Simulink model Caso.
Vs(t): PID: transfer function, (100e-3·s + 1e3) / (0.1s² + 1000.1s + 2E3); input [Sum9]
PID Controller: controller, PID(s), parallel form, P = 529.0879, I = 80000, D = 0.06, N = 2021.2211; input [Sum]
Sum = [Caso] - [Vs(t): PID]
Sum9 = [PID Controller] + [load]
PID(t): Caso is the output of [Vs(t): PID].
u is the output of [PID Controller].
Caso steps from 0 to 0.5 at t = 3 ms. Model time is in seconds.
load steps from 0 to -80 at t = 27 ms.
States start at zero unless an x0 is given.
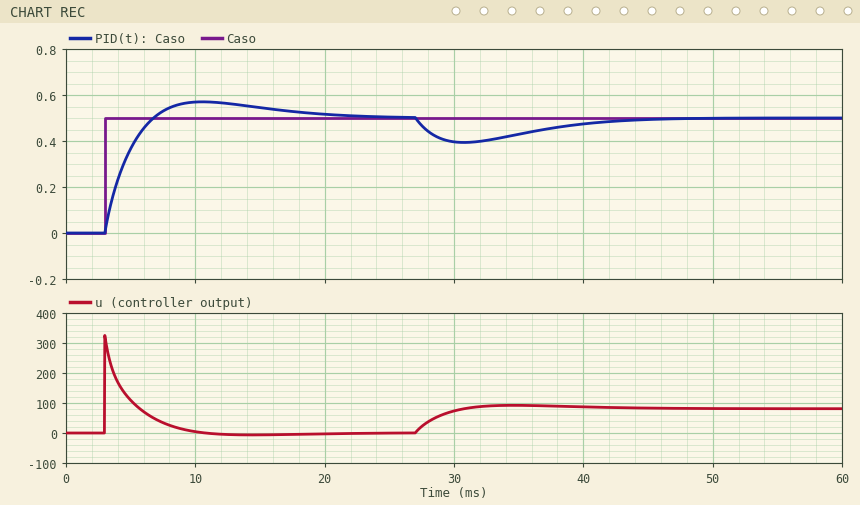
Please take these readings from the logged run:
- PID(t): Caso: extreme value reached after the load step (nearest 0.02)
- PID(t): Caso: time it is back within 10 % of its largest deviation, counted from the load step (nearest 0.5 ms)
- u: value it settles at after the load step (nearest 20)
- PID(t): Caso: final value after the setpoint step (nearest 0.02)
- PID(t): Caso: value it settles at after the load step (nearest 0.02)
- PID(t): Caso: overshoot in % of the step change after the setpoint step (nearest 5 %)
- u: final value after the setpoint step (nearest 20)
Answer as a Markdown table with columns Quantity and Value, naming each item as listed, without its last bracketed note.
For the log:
| Quantity | Value |
|---|---|
| PID(t): Caso: extreme value reached after the load step | 0.40 |
| PID(t): Caso: time it is back within 10 % of its largest deviation, counted from the load step | 16.5 ms |
| u: value it settles at after the load step | 80 |
| PID(t): Caso: final value after the setpoint step | 0.50 |
| PID(t): Caso: value it settles at after the load step | 0.50 |
| PID(t): Caso: overshoot in % of the step change after the setpoint step | 15 % |
| u: final value after the setpoint step | 0 |
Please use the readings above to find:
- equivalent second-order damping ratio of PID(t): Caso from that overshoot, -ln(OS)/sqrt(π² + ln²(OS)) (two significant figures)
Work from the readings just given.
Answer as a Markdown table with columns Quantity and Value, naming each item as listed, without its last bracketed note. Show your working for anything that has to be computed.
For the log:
| Quantity | Value |
|---|---|
| equivalent second-order damping ratio of PID(t): Caso from that overshoot, -ln(OS)/sqrt(π² + ln²(OS)) | ln(0.15) = -1.897; 1.897 / sqrt(9.870 + 3.599) = 0.52 |
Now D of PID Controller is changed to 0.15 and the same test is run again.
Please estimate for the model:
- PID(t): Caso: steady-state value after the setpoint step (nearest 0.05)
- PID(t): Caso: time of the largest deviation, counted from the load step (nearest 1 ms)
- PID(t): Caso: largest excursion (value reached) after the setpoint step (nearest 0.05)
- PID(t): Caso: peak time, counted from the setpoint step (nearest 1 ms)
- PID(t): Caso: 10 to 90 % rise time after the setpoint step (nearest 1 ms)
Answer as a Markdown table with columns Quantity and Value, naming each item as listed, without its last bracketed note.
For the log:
| Quantity | Value |
|---|---|
| PID(t): Caso: steady-state value after the setpoint step | 0.50 |
| PID(t): Caso: time of the largest deviation, counted from the load step | 4 ms |
| PID(t): Caso: largest excursion (value reached) after the setpoint step | 0.55 |
| PID(t): Caso: peak time, counted from the setpoint step | 8 ms |
| PID(t): Caso: 10 to 90 % rise time after the setpoint step | 3 ms |
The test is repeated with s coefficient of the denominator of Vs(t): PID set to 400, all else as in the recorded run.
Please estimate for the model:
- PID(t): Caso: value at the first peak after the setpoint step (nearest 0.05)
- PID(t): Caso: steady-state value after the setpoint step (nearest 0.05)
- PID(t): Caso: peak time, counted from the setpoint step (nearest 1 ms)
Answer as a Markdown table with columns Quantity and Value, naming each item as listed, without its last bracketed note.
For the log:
| Quantity | Value |
|---|---|
| PID(t): Caso: value at the first peak after the setpoint step | 0.55 |
| PID(t): Caso: steady-state value after the setpoint step | 0.50 |
| PID(t): Caso: peak time, counted from the setpoint step | 4 ms |
